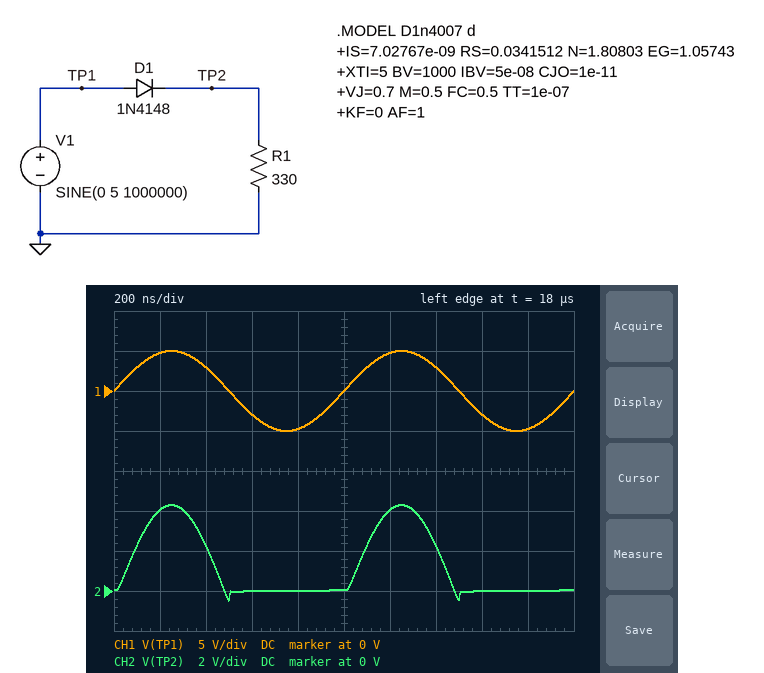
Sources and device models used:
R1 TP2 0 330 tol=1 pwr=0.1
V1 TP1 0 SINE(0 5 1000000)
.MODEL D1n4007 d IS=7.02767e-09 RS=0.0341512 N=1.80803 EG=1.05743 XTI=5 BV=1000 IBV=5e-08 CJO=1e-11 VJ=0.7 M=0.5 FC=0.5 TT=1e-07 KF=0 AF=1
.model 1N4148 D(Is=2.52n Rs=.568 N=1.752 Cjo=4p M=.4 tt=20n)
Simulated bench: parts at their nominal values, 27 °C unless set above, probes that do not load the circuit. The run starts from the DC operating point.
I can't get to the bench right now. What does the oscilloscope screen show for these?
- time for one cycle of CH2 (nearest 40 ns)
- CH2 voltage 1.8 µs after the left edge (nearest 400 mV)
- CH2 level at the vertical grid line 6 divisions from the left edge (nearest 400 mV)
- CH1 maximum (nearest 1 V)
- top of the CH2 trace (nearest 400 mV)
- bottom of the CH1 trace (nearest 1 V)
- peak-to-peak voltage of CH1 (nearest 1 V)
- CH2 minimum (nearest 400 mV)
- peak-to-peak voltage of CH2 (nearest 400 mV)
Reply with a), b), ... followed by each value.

a) 1.00 µs
b) 0 V
c) 4.0 V
d) 5 V
e) 4.4 V
f) -5 V
g) 10 V
h) -400 mV
i) 4.8 V
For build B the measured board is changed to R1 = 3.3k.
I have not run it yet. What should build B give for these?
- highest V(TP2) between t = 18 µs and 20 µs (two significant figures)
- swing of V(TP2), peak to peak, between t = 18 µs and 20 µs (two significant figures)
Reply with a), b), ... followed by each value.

a) 4.4 V
b) 5.0 V
